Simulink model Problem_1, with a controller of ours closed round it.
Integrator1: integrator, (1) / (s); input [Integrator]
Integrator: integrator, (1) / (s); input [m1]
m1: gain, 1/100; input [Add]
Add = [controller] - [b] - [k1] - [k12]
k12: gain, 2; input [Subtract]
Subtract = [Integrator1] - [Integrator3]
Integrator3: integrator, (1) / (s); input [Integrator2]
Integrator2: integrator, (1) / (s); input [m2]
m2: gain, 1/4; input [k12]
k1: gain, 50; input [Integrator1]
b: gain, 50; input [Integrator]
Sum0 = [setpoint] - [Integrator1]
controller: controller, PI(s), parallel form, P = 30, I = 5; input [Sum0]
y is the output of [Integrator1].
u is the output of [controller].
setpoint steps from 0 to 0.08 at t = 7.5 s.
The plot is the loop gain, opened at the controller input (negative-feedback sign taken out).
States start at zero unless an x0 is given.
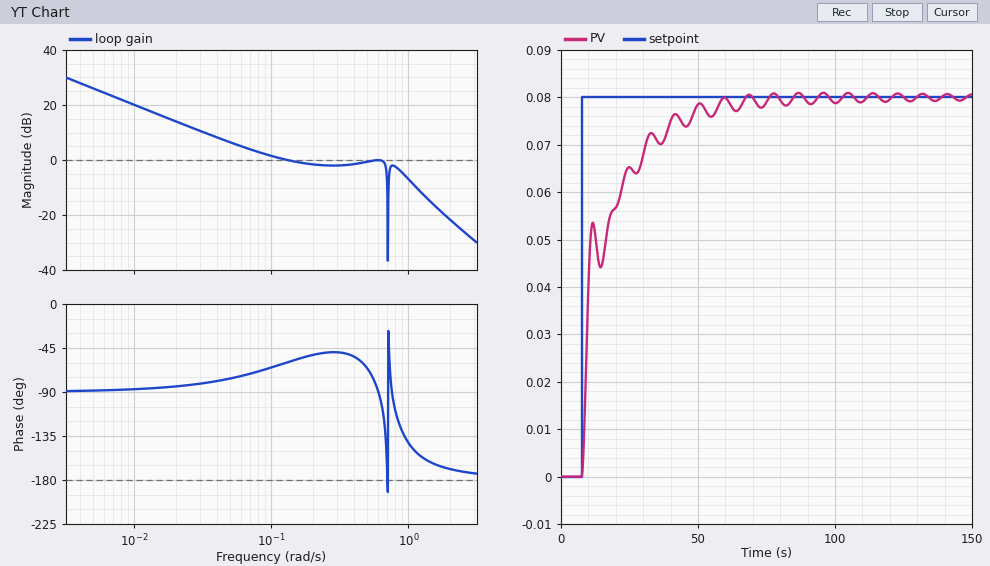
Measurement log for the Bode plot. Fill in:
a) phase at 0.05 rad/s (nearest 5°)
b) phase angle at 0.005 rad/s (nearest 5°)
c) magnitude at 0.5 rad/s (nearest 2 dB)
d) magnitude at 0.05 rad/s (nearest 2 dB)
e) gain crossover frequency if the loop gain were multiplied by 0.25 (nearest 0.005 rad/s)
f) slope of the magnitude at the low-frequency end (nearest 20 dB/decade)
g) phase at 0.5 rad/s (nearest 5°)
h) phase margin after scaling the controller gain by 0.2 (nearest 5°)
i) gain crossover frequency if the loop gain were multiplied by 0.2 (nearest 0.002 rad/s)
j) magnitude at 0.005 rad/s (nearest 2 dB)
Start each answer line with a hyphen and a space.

- -75°
- -90°
- 0 dB
- 6 dB
- 0.025 rad/s
- -20 dB/decade
- -65°
- 95°
- 0.020 rad/s
- 26 dB
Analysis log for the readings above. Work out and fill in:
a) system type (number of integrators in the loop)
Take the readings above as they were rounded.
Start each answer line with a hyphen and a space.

- 1
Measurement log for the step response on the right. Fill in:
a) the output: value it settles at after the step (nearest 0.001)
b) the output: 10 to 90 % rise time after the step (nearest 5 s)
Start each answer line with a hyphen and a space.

- 0.080
- 25 s
